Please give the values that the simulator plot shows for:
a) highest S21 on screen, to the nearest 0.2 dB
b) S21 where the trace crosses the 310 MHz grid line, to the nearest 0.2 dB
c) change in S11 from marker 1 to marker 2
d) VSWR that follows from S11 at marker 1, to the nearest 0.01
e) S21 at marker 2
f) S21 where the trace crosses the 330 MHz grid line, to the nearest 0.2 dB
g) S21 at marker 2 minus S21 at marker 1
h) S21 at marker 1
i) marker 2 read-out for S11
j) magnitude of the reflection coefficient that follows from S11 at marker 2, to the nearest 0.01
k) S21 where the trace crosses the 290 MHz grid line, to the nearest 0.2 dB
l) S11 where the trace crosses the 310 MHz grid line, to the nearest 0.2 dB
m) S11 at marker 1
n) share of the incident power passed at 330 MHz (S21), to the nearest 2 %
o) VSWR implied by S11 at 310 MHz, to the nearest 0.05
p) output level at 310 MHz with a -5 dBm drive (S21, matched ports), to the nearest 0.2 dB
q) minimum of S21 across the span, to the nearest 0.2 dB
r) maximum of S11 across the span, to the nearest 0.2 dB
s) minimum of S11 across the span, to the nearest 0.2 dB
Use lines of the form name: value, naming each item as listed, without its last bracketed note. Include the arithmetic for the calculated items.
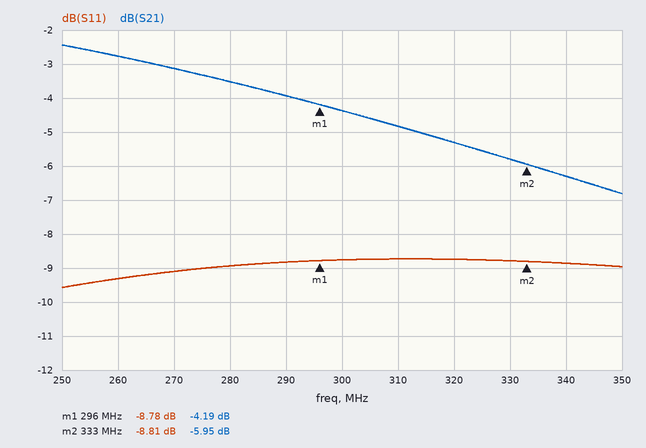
highest S21 on screen, to the nearest 0.2 dB: -2.4 dB
S21 where the trace crosses the 310 MHz grid line, to the nearest 0.2 dB: -4.8 dB
change in S11 from marker 1 to marker 2: -8.81 − (-8.78) = -0.03 dB
VSWR that follows from S11 at marker 1, to the nearest 0.01: (1 + 0.3639)/(1 − 0.3639) ≈ 2.14
S21 at marker 2: -5.95 dB
S21 where the trace crosses the 330 MHz grid line, to the nearest 0.2 dB: -5.8 dB
S21 at marker 2 minus S21 at marker 1: -5.95 − (-4.19) = -1.76 dB
S21 at marker 1: -4.19 dB
marker 2 read-out for S11: -8.81 dB
magnitude of the reflection coefficient that follows from S11 at marker 2, to the nearest 0.01: 10^(-8.81/20) ≈ 0.36
S21 where the trace crosses the 290 MHz grid line, to the nearest 0.2 dB: -4.0 dB
S11 where the trace crosses the 310 MHz grid line, to the nearest 0.2 dB: -8.8 dB
S11 at marker 1: -8.78 dB
share of the incident power passed at 330 MHz (S21), to the nearest 2 %: 10^(-5.8/10) ≈ 26 %
VSWR implied by S11 at 310 MHz, to the nearest 0.05: |Γ| = 10^(-8.8/20) = 0.3631; VSWR = (1 + 0.3631)/(1 − 0.3631) ≈ 2.14, so 2.15 to the nearest 0.05
output level at 310 MHz with a -5 dBm drive (S21, matched ports), to the nearest 0.2 dB: -5 dBm + (-4.8 dB) = -9.8 dBm
minimum of S21 across the span, to the nearest 0.2 dB: -6.8 dB
maximum of S11 across the span, to the nearest 0.2 dB: -8.8 dB
minimum of S11 across the span, to the nearest 0.2 dB: -9.6 dB
